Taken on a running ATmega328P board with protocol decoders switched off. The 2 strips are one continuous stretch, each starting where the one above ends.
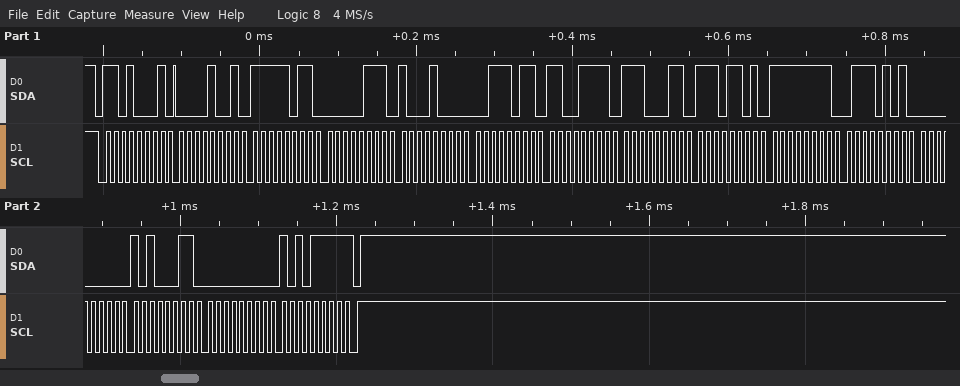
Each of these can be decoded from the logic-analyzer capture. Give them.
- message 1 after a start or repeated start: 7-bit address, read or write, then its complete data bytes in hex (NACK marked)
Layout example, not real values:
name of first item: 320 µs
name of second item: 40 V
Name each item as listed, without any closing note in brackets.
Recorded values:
message 1 after a start or repeated start: 7-bit address, read or write, then its complete data bytes in hex: 0x68 read: 09 FB 07 88 3B CF E3 ED FF 75 00 A3 00 AF NACK
